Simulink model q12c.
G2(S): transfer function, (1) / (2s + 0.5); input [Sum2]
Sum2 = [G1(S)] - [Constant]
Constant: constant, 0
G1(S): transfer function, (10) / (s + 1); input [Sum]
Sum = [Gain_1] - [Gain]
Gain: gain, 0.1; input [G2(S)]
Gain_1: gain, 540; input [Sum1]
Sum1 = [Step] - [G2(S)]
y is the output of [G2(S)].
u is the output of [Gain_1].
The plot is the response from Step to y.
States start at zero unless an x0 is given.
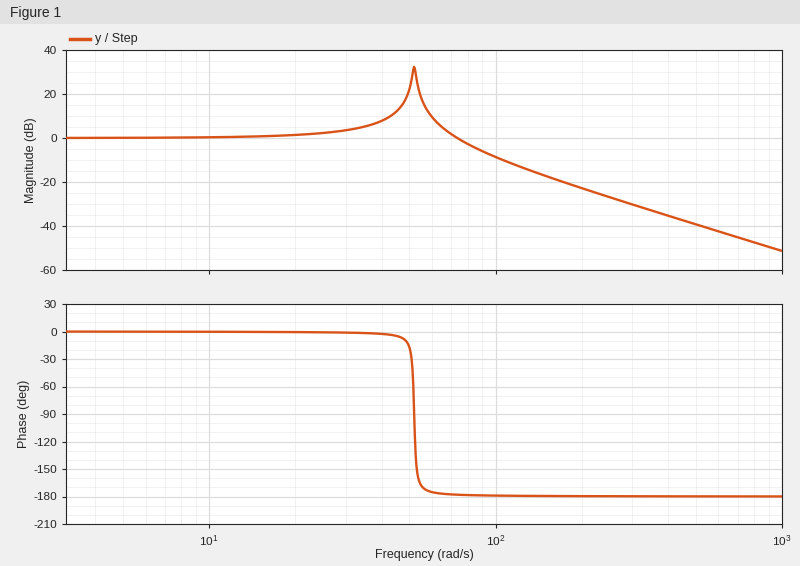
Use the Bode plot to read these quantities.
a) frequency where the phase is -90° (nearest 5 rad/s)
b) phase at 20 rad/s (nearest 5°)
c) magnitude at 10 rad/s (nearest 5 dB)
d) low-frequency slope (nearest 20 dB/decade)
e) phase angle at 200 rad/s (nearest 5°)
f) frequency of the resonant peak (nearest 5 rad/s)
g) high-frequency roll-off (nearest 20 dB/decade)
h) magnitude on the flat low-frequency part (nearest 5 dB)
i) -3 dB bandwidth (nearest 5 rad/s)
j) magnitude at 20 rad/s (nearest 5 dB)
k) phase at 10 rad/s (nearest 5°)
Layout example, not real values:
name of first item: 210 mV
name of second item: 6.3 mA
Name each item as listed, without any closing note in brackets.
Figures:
frequency where the phase is -90°: 50 rad/s
phase at 20 rad/s: 0°
magnitude at 10 rad/s: 0 dB
low-frequency slope: 0 dB/decade
phase angle at 200 rad/s: -180°
frequency of the resonant peak: 50 rad/s
high-frequency roll-off: -40 dB/decade
magnitude on the flat low-frequency part: 0 dB
-3 dB bandwidth: 80 rad/s
magnitude at 20 rad/s: 0 dB
phase at 10 rad/s: 0°
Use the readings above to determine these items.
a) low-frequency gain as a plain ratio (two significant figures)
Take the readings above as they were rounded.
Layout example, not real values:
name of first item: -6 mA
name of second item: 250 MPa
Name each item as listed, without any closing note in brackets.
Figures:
low-frequency gain as a plain ratio: 1.0
